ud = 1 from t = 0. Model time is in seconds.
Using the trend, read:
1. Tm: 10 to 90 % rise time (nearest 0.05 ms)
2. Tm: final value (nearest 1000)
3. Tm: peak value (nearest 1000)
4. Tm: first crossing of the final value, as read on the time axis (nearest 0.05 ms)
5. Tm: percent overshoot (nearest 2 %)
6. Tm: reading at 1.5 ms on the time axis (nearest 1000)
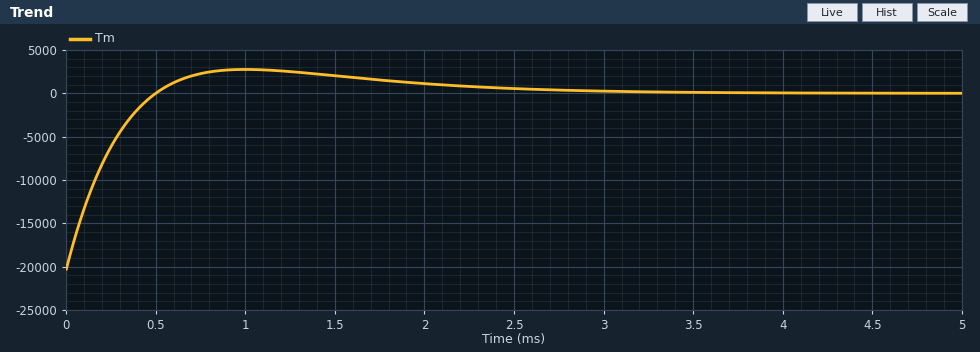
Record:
0.35 ms
0
3000
0.50 ms
14 %
2000
